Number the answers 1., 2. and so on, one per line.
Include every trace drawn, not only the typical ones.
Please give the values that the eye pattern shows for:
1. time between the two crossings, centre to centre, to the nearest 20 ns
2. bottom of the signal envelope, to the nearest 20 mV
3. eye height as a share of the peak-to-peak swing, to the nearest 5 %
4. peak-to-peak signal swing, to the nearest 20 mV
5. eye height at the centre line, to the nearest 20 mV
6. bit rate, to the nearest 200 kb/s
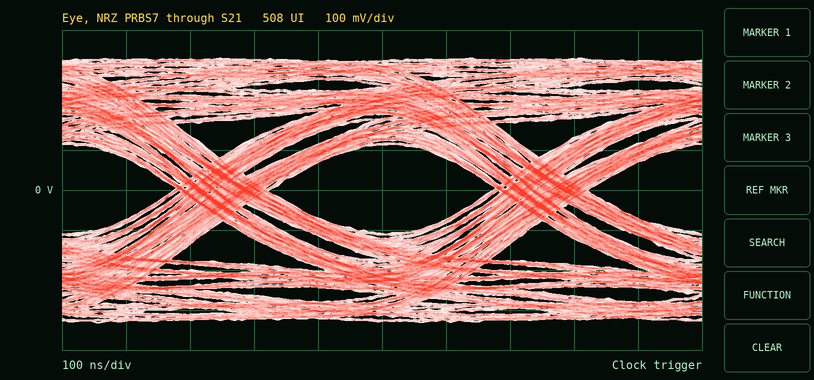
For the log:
1. 500 ns
2. -340 mV
3. 35 %
4. 660 mV
5. 220 mV
6. 2.0 Mb/s
